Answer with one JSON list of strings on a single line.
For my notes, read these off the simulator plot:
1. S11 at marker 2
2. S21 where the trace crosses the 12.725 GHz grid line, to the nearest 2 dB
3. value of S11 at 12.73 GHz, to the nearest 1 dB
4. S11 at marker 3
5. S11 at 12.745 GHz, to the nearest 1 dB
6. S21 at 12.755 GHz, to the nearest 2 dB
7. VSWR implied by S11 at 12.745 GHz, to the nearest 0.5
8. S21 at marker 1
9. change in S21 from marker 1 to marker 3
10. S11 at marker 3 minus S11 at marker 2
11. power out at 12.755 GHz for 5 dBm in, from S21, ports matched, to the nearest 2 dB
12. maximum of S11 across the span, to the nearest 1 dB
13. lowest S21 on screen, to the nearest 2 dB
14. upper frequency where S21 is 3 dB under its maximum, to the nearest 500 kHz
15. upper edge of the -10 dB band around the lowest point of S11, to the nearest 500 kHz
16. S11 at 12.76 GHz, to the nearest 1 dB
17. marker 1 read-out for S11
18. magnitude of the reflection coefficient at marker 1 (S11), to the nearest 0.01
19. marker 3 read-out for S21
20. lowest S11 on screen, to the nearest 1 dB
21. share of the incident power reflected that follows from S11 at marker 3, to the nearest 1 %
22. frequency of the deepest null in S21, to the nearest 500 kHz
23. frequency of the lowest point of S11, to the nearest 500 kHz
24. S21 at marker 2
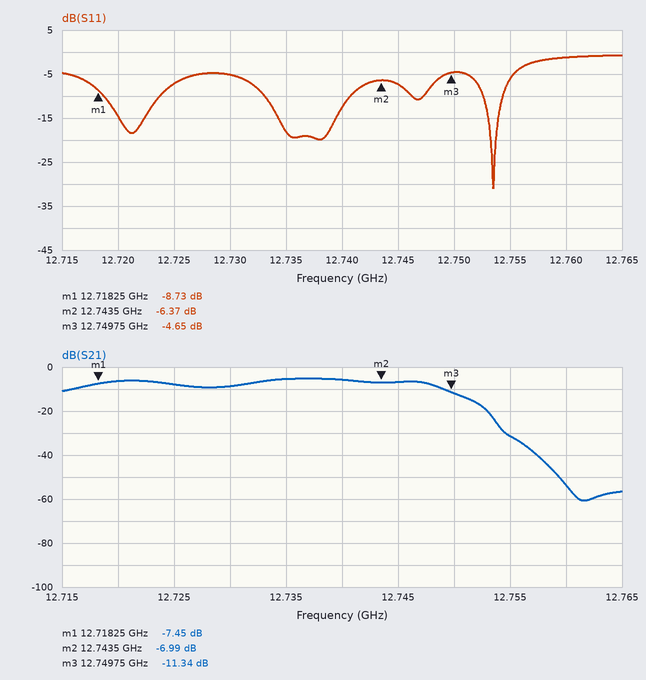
["-6.37 dB", "-8 dB", "-5 dB", "-4.65 dB", "-7 dB", "-32 dB", "2.5", "-7.45 dB", "-3.89 dB", "1.72 dB", "-26 dBm", "-1 dB", "-60 dB", "12.7480 GHz", "12.7545 GHz", "-1 dB", "-8.73 dB", "0.37", "-11.34 dB", "-31 dB", "34 %", "12.7615 GHz", "12.7535 GHz", "-6.99 dB"]
